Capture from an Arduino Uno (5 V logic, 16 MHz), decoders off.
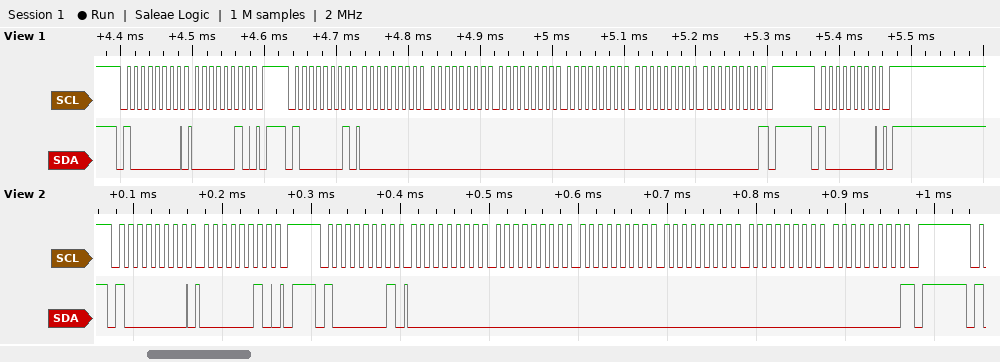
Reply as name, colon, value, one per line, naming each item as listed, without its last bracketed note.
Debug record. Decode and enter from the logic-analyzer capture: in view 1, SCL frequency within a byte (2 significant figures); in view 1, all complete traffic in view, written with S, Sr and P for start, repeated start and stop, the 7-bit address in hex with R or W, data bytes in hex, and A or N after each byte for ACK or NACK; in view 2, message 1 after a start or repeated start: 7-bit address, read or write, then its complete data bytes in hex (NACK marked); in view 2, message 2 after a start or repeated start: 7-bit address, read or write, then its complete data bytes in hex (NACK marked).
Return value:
in view 1, SCL frequency within a byte: 100 kHz
in view 1, all complete traffic in view, written with S, Sr and P for start, repeated start and stop, the 7-bit address in hex with R or W, data bytes in hex, and A or N after each byte for ACK or NACK: S 40W A 02 A P S 40R A 00 A 00 A 00 A 00 A 00 A 00 N P S 40W A P
in view 2, message 1 after a start or repeated start: 7-bit address, read or write, then its complete data bytes in hex: 0x40 write: 02
in view 2, message 2 after a start or repeated start: 7-bit address, read or write, then its complete data bytes in hex: 0x40 read: 00 00 00 00 00 00 NACK
